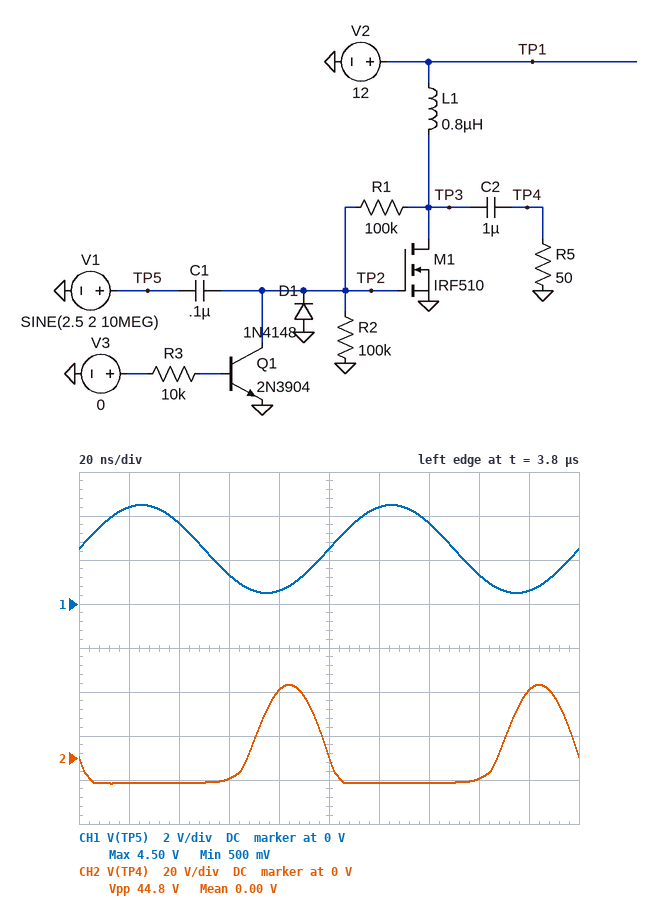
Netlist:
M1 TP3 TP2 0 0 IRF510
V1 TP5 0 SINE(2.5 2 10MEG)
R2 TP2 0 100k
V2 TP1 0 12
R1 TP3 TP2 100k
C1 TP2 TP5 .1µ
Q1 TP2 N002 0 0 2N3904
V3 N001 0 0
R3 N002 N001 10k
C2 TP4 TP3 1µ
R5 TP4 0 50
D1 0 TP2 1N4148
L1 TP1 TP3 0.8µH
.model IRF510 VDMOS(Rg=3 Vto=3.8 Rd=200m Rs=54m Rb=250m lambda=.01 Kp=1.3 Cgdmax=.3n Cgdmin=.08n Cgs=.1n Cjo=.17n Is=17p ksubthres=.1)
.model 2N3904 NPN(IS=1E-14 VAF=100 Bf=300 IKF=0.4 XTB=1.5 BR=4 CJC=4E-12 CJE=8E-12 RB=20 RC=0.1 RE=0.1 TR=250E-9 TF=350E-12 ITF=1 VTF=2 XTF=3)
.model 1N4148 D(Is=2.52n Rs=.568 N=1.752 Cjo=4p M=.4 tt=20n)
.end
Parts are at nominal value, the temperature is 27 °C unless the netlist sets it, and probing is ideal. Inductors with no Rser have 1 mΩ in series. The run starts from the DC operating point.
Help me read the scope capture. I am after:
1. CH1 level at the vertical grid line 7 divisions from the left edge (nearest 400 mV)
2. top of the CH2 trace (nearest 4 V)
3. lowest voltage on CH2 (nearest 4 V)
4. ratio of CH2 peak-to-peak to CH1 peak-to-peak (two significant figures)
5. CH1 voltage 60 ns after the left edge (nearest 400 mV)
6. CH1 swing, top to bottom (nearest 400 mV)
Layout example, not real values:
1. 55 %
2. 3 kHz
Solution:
1. 3.6 V
2. 32 V
3. -12 V
4. 11
5. 1.2 V
6. 4.0 V
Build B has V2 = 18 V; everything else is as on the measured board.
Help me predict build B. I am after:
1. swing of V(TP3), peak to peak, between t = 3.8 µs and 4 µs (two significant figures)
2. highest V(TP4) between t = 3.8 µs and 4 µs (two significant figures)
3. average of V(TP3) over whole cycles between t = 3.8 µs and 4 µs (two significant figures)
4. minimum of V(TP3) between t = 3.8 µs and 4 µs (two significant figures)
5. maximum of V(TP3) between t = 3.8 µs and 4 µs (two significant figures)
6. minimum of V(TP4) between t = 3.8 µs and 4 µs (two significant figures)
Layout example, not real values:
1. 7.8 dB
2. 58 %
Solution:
1. 51 V
2. 37 V
3. 18 V
4. 4.0 V
5. 55 V
6. -14 V
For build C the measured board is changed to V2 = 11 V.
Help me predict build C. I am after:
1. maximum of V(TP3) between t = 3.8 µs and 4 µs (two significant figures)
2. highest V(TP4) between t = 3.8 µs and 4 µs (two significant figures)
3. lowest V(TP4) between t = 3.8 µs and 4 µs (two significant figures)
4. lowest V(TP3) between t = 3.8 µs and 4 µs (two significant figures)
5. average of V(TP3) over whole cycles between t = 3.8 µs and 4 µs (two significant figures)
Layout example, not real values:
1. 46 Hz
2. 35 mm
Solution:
1. 40 V
2. 29 V
3. -11 V
4. 260 mV
5. 11 V
